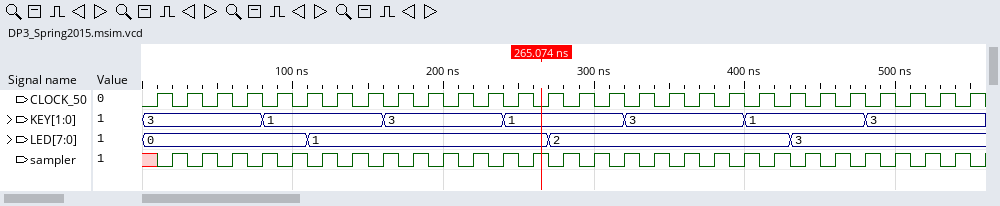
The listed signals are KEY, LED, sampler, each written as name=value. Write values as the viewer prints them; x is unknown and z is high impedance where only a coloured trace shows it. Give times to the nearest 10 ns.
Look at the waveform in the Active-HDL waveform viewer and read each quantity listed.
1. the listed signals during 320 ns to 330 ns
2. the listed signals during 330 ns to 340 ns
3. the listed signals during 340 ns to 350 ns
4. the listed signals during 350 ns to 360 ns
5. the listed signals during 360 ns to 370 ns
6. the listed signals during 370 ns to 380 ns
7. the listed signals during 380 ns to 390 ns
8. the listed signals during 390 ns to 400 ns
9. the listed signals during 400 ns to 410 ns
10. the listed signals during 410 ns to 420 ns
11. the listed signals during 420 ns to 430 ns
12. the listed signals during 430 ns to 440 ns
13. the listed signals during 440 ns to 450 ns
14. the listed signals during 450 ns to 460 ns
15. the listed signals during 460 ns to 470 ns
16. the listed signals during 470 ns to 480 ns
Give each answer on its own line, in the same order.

KEY=3, LED=2, sampler=1
KEY=3, LED=2, sampler=0
KEY=3, LED=2, sampler=1
KEY=3, LED=2, sampler=0
KEY=3, LED=2, sampler=1
KEY=3, LED=2, sampler=0
KEY=3, LED=2, sampler=1
KEY=3, LED=2, sampler=0
KEY=1, LED=2, sampler=1
KEY=1, LED=2, sampler=0
KEY=1, LED=2, sampler=1
KEY=1, LED=3, sampler=0
KEY=1, LED=3, sampler=1
KEY=1, LED=3, sampler=0
KEY=1, LED=3, sampler=1
KEY=1, LED=3, sampler=0
